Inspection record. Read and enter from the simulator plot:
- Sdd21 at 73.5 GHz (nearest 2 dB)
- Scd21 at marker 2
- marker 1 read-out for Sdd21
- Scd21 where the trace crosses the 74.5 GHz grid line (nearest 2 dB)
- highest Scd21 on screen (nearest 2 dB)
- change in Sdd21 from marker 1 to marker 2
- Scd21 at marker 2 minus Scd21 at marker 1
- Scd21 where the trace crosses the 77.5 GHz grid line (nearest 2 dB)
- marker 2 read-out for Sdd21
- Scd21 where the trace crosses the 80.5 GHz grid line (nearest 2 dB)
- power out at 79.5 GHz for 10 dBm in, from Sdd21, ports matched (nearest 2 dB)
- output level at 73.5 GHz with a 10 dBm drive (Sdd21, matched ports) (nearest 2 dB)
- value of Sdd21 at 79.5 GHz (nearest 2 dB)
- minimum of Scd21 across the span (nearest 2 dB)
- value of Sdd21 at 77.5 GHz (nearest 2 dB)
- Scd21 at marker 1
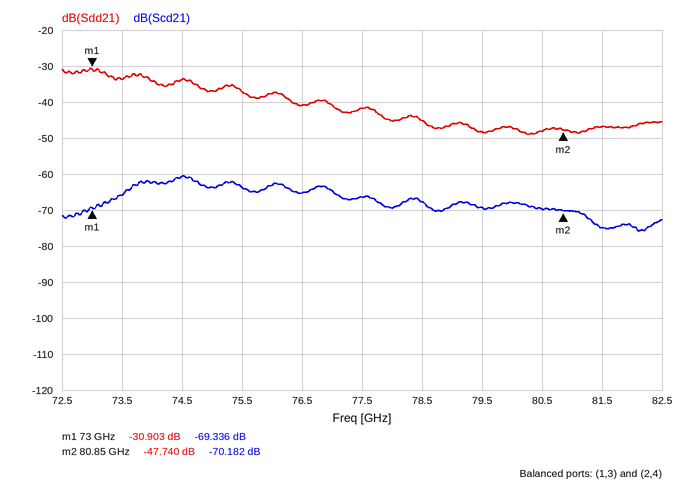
-34 dB
-70.182 dB
-30.903 dB
-60 dB
-60 dB
-16.837 dB
-0.846 dB
-66 dB
-47.740 dB
-70 dB
-38 dBm
-24 dBm
-48 dB
-76 dB
-42 dB
-69.336 dB
